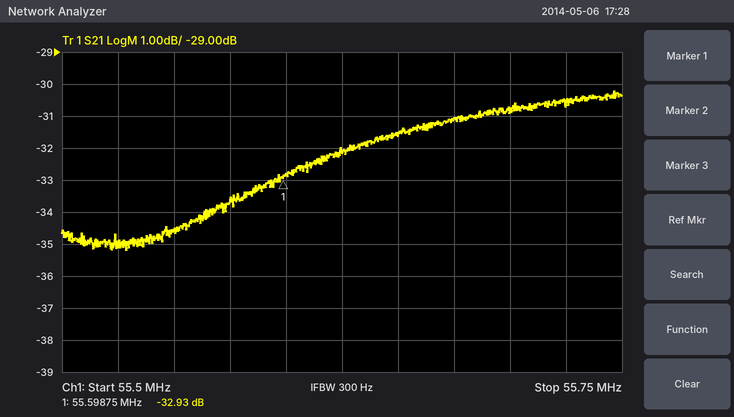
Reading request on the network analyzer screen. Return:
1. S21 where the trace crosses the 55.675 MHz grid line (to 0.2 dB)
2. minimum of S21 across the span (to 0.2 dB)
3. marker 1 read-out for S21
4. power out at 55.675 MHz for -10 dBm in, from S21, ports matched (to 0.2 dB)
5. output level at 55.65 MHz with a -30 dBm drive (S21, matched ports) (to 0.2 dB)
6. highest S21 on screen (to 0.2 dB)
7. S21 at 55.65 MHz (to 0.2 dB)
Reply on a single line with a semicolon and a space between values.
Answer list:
-31.0 dB; -35.2 dB; -32.93 dB; -41.0 dBm; -61.6 dBm; -30.2 dB; -31.6 dB
